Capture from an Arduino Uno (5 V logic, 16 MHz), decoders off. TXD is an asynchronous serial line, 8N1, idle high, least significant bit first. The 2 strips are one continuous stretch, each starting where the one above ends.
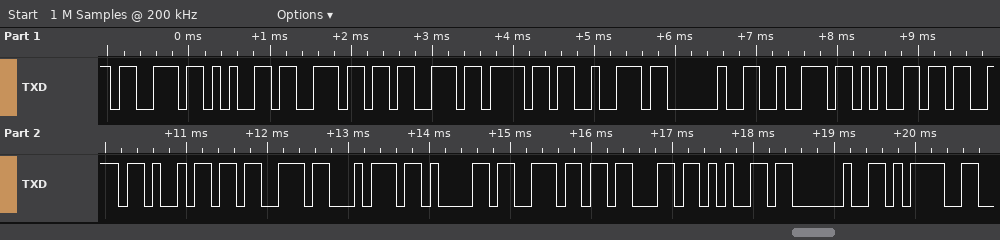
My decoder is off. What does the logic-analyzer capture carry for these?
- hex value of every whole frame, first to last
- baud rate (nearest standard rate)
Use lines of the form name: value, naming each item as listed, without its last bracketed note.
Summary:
hex value of every whole frame, first to last: 73 65 6E 73 6F 72 20 72 65 73 69 73 74 61 6E 63 65 20 3D
baud rate: 9600 baud
